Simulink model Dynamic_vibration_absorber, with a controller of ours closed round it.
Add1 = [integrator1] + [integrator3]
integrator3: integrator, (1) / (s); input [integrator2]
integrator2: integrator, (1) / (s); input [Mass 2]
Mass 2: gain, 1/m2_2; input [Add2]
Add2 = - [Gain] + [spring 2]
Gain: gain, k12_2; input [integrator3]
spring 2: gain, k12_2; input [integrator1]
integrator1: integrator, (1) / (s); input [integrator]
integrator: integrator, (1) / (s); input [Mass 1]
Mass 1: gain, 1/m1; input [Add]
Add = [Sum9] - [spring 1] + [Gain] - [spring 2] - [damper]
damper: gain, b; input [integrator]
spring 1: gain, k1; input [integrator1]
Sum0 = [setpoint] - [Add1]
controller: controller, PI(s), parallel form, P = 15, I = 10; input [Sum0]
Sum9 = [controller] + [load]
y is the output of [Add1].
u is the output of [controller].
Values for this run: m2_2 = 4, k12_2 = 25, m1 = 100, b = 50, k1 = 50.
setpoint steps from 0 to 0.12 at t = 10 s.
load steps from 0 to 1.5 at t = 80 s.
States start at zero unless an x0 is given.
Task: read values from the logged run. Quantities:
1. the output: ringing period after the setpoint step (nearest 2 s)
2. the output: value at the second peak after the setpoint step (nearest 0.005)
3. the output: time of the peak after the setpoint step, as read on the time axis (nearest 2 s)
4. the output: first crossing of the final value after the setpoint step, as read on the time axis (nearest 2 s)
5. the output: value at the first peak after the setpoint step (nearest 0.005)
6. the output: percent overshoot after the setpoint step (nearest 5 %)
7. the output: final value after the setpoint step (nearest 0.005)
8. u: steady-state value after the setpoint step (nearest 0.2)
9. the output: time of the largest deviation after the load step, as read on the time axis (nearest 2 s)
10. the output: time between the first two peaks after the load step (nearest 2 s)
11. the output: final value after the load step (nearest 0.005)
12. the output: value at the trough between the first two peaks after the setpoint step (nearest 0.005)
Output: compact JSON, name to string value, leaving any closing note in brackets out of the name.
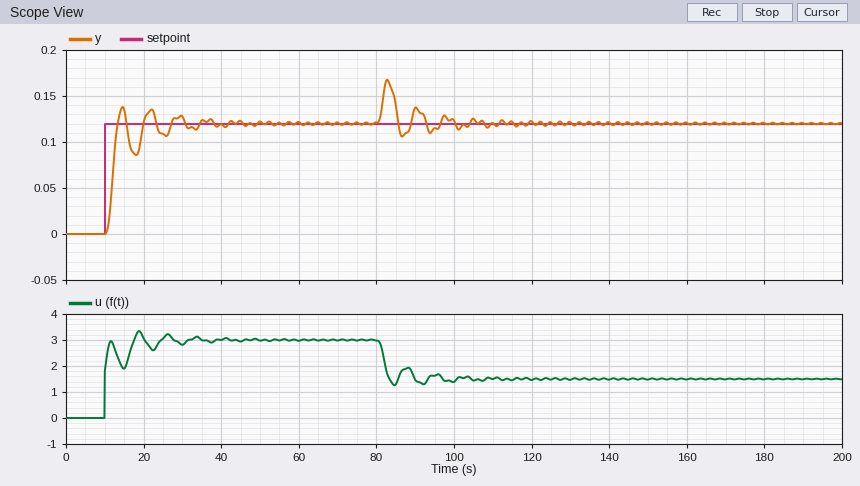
{"the output: ringing period after the setpoint step": "8 s", "the output: value at the second peak after the setpoint step": "0.135", "the output: time of the peak after the setpoint step, as read on the time axis": "14 s", "the output: first crossing of the final value after the setpoint step, as read on the time axis": "14 s", "the output: value at the first peak after the setpoint step": "0.140", "the output: percent overshoot after the setpoint step": "15 %", "the output: final value after the setpoint step": "0.120", "u: steady-state value after the setpoint step": "3.0", "the output: time of the largest deviation after the load step, as read on the time axis": "82 s", "the output: time between the first two peaks after the load step": "8 s", "the output: final value after the load step": "0.120", "the output: value at the trough between the first two peaks after the setpoint step": "0.085"}
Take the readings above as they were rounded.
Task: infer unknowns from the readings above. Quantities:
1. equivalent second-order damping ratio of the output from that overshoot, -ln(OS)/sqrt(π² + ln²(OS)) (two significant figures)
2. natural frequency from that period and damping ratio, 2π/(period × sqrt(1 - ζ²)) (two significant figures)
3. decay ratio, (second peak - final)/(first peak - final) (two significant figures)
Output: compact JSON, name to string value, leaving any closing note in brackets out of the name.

{"equivalent second-order damping ratio of the output from that overshoot, -ln(OS)/sqrt(π² + ln²(OS))": "0.52", "natural frequency from that period and damping ratio, 2π/(period × sqrt(1 - ζ²))": "0.92 rad/s", "decay ratio, (second peak - final)/(first peak - final)": "0.75"}
